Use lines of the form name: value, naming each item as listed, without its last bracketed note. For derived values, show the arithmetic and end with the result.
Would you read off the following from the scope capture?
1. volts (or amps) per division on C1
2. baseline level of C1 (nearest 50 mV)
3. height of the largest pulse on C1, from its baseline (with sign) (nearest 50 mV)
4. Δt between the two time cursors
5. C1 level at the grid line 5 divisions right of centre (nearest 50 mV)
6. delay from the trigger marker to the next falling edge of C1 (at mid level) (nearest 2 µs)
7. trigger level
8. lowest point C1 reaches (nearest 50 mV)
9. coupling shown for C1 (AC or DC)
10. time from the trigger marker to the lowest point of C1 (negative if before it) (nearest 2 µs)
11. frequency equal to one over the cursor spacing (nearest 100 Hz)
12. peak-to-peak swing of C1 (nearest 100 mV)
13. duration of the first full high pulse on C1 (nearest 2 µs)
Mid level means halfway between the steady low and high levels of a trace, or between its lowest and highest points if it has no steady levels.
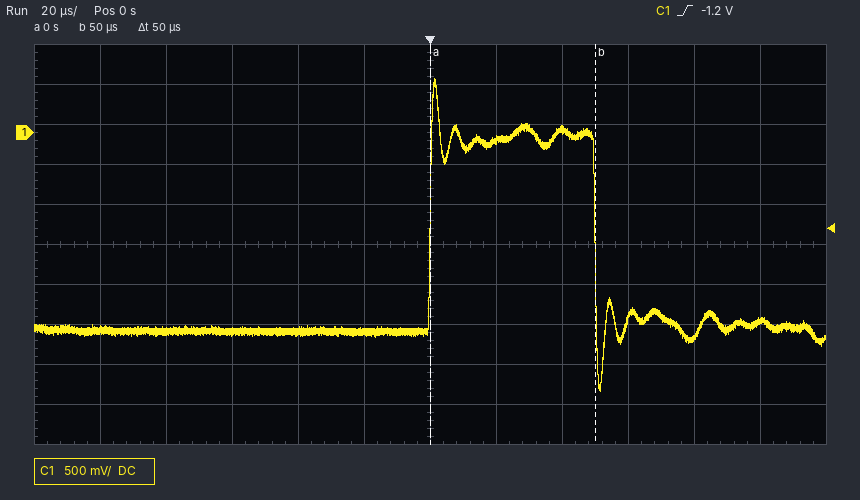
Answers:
volts (or amps) per division on C1: 500 mV
baseline level of C1: -2.50 V
height of the largest pulse on C1, from its baseline (with sign): +3.15 V
Δt between the two time cursors: 50 µs
C1 level at the grid line 5 divisions right of centre: -2.35 V
delay from the trigger marker to the next falling edge of C1 (at mid level): 50 µs
trigger level: -1.2 V
lowest point C1 reaches: -3.25 V
coupling shown for C1: DC
time from the trigger marker to the lowest point of C1 (negative if before it): +52 µs
frequency equal to one over the cursor spacing: 1 / 50 µs ≈ 20.0 kHz
peak-to-peak swing of C1: 3.90 V
duration of the first full high pulse on C1: 50 µs
